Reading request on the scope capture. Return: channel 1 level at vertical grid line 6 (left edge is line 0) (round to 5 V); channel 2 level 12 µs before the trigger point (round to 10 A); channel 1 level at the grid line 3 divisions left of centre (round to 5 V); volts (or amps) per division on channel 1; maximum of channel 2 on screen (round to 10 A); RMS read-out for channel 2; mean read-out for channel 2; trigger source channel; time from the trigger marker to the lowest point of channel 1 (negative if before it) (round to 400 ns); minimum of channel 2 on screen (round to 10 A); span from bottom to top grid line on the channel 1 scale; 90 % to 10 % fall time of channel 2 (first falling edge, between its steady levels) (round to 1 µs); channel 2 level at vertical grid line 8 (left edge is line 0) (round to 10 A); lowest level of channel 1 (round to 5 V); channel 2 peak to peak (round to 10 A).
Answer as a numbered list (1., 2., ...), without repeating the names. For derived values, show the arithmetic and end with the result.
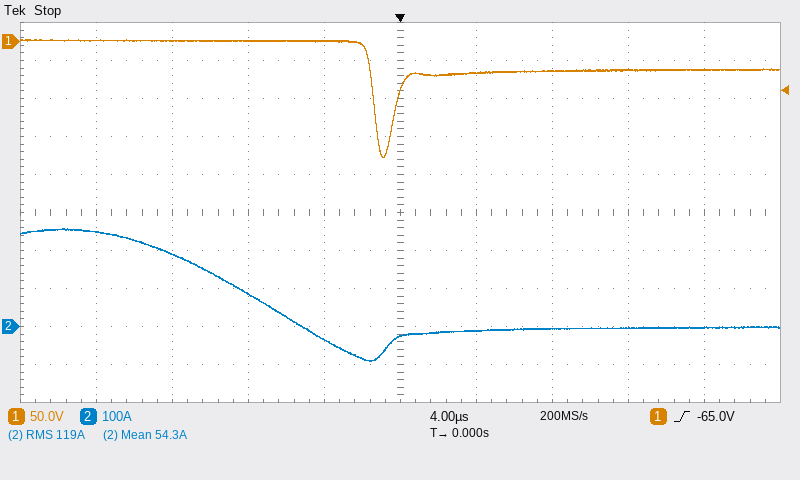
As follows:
1. -40 V
2. 190 A
3. 0 V
4. 50 V
5. 260 A
6. 119 A
7. 54.3 A
8. channel 1
9. -800 ns
10. -90 A
11. 500 V
12. 8 µs
13. 0 A
14. -155 V
15. 260 A − (-90 A) = 350 A
